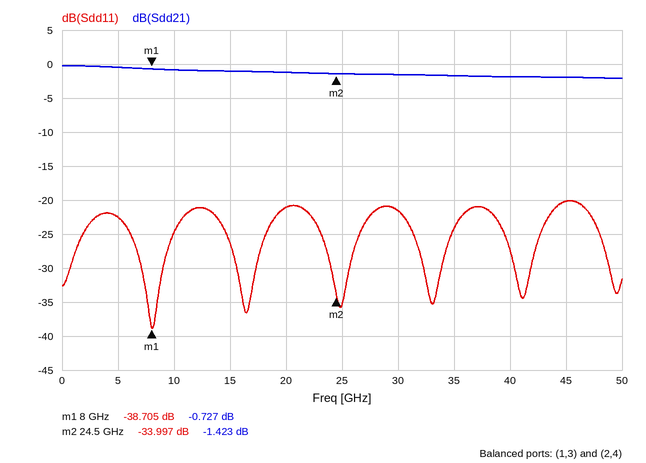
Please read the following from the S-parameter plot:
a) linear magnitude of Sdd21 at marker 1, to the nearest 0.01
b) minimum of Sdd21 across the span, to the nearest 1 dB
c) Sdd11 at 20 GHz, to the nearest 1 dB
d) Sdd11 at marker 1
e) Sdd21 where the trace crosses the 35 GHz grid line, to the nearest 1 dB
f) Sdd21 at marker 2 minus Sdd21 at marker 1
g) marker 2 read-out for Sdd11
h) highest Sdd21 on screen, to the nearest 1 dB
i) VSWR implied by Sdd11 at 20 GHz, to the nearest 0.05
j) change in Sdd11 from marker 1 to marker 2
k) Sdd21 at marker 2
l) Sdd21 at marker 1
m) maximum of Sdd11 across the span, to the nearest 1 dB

0.92
-2 dB
-21 dB
-38.705 dB
-2 dB
-0.696 dB
-33.997 dB
0 dB
1.20
4.708 dB
-1.423 dB
-0.727 dB
-20 dB
